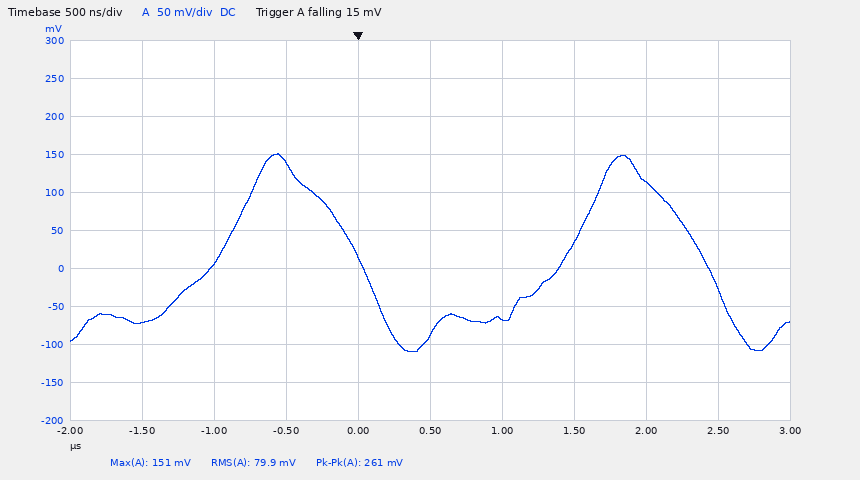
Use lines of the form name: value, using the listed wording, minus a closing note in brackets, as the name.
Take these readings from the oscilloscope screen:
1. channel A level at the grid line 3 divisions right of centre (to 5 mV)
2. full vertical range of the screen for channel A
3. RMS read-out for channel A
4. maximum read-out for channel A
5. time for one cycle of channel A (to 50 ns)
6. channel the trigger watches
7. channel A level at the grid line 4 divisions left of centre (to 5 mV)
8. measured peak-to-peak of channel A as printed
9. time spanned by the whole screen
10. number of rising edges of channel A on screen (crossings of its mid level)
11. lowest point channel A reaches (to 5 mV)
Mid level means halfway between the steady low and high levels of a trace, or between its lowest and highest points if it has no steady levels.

channel A level at the grid line 3 divisions right of centre: 115 mV
full vertical range of the screen for channel A: 500 mV
RMS read-out for channel A: 79.9 mV
maximum read-out for channel A: 151 mV
time for one cycle of channel A: 2.40 µs
channel the trigger watches: channel A
channel A level at the grid line 4 divisions left of centre: -70 mV
measured peak-to-peak of channel A as printed: 261 mV
time spanned by the whole screen: 5 µs
number of rising edges of channel A on screen: 2
lowest point channel A reaches: -110 mV
